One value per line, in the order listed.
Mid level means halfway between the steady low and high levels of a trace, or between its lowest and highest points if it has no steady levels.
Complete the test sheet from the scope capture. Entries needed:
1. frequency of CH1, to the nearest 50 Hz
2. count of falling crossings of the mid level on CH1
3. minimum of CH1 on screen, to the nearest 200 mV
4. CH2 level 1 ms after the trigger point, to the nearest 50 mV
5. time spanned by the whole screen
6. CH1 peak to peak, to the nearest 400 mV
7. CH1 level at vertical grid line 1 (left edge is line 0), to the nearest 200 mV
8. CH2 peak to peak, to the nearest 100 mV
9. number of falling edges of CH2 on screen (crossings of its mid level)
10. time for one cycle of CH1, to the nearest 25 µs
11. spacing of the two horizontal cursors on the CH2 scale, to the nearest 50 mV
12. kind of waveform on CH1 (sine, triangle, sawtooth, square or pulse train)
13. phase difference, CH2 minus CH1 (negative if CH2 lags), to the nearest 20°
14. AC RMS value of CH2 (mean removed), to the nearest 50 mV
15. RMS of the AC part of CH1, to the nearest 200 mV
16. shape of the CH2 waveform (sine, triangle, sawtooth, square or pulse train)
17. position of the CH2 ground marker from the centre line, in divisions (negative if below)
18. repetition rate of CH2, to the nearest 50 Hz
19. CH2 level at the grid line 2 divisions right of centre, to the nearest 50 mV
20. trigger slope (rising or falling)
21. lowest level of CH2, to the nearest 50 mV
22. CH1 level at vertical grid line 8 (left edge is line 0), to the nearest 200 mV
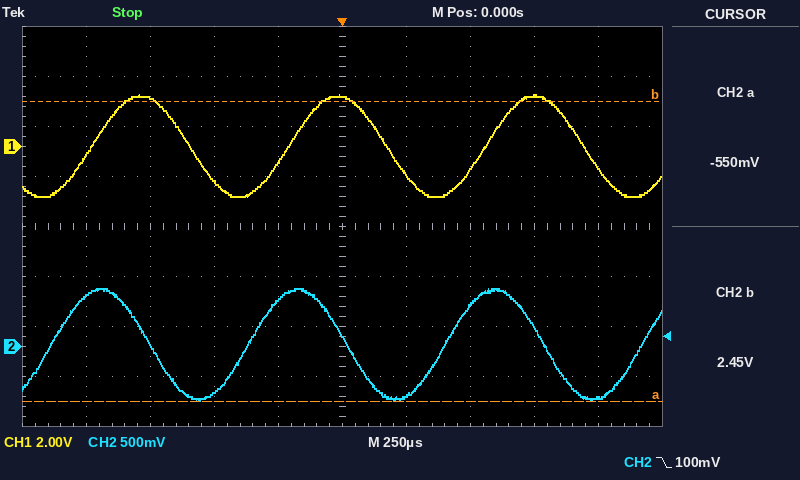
1.30 kHz
3
-2.0 V
-500 mV
2.5 ms
4.0 V
-400 mV
1.10 V
3
775 µs
3.00 V
sine
+80°
400 mV
1.4 V
sine
-2.4 div
1.30 kHz
400 mV
falling
-550 mV
2.0 V
